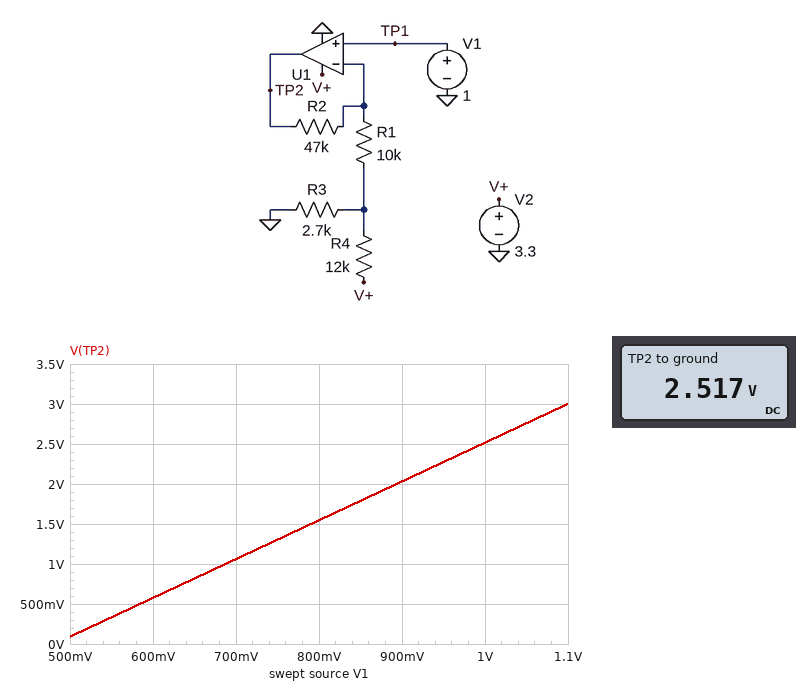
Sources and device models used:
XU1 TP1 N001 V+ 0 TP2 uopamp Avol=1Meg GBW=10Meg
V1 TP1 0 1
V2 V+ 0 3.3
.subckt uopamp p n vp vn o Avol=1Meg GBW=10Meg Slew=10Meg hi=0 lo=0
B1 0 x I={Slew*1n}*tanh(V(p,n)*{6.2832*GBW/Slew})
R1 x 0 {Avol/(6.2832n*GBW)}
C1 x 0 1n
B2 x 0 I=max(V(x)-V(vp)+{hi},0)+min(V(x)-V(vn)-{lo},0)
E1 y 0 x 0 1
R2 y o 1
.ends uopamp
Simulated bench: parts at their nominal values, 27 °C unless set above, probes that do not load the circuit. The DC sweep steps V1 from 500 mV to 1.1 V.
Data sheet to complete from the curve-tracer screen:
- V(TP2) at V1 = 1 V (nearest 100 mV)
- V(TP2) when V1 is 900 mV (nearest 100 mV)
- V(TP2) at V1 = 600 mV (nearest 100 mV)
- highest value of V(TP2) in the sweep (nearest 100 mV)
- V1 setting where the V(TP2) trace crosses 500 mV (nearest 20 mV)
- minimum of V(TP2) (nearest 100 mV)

2.5 V
2.0 V
600 mV
3.0 V
580 mV
100 mV
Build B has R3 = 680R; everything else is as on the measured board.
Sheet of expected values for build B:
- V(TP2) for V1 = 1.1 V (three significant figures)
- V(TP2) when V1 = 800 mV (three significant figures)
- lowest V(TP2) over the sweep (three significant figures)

3.31 V
3.30 V
1.93 V
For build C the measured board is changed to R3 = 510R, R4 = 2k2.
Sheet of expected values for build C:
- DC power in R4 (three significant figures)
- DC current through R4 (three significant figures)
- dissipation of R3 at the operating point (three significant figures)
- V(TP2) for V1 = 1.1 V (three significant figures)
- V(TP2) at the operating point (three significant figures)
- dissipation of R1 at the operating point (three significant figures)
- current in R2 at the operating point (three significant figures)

3.23 mW
1.21 mA
793 µW
3.26 V
2.71 V
13.2 µW
36.4 µA
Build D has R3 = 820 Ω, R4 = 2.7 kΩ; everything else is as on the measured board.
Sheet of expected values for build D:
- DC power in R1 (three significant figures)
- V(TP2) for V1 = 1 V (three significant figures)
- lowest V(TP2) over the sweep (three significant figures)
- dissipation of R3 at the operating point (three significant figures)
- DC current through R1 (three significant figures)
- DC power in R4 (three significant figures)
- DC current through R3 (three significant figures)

4.73 µW
2.02 V
-6.57 mV
747 µW
21.8 µA
2.35 mW
954 µA
